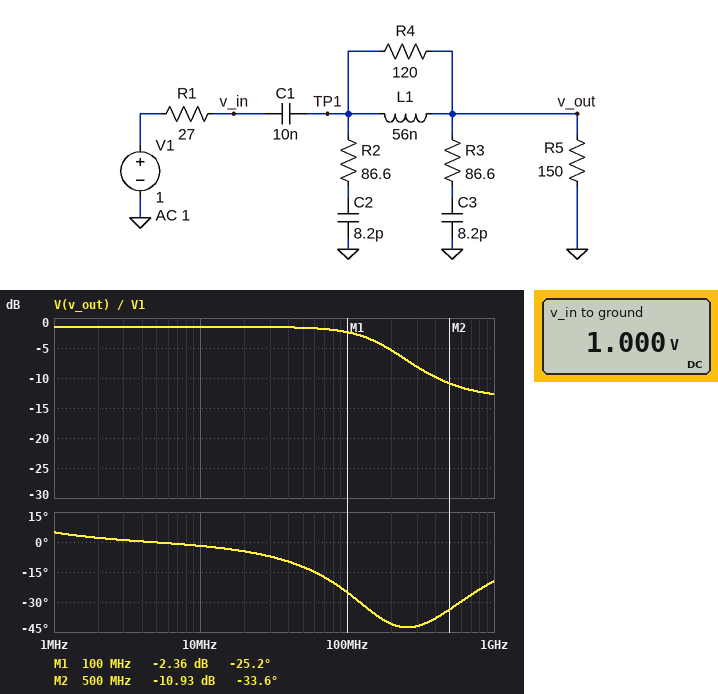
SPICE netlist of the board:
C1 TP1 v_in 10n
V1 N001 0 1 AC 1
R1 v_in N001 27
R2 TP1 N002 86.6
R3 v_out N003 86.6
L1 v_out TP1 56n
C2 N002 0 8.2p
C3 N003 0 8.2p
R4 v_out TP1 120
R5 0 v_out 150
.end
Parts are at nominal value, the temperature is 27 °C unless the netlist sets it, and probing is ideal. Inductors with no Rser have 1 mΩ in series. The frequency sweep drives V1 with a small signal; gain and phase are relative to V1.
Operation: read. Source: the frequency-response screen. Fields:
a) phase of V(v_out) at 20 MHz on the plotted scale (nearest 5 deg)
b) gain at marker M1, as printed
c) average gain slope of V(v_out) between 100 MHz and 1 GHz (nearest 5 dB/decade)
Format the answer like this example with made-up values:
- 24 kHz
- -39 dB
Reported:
- -5 deg
- -2.36 dB
- -10 dB/decade
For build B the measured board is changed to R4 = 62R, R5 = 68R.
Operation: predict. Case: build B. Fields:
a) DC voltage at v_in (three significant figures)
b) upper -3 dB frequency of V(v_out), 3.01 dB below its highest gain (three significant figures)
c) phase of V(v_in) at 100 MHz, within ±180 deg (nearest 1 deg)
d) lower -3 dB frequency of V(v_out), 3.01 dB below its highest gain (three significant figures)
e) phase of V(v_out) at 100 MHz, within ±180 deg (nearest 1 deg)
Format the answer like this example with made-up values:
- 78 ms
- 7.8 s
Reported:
- 1.00 V
- 129 MHz
- -2 deg
- 167 kHz
- -26 deg
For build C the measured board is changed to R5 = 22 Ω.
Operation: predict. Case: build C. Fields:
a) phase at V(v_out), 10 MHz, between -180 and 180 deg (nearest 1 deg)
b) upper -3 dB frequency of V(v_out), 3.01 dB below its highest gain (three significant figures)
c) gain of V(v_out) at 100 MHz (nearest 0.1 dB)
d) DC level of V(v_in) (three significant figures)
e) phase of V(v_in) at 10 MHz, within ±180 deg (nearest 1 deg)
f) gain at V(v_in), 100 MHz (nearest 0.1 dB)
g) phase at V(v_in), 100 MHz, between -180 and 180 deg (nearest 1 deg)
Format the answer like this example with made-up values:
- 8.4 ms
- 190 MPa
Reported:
- -3 deg
- 101 MHz
- -9.9 dB
- 1.00 V
- 2 deg
- -3.7 dB
- 12 deg
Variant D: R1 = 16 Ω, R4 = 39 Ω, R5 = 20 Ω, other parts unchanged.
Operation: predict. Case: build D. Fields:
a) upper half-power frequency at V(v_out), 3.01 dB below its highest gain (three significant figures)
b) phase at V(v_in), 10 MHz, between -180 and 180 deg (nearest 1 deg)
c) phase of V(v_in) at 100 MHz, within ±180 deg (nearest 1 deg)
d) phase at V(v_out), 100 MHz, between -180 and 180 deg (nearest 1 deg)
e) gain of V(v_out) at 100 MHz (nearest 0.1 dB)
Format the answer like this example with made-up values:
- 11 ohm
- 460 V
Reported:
- 71.0 MHz
- 2 deg
- 4 deg
- -26 deg
- -9.4 dB
